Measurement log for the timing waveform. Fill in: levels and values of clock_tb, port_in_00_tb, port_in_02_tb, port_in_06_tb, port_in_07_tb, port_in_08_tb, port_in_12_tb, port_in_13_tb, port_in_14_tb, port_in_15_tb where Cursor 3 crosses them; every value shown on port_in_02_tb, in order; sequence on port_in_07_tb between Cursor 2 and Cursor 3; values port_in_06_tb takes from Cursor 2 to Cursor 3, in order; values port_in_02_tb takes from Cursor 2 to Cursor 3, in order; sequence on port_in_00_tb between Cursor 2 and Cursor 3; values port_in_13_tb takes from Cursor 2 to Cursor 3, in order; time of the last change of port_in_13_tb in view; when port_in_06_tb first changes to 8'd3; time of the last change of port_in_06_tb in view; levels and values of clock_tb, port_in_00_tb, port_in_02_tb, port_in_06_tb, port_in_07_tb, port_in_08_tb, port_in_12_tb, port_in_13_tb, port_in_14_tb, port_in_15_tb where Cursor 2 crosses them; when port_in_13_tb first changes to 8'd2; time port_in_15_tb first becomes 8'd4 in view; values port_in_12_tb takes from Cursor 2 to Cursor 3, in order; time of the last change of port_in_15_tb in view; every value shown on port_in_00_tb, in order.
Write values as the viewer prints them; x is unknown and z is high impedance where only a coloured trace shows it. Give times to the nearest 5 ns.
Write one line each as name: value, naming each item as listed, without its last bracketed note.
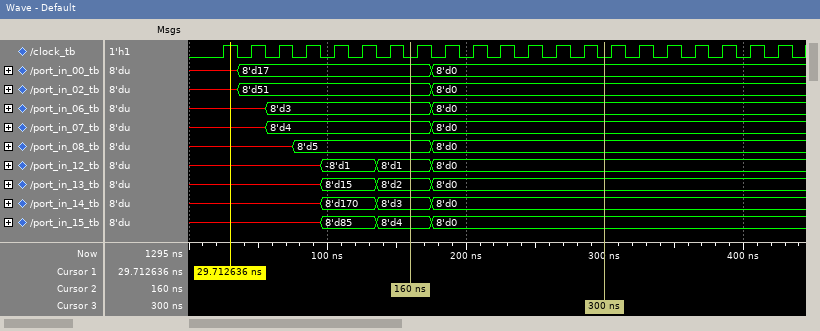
levels and values of clock_tb, port_in_00_tb, port_in_02_tb, port_in_06_tb, port_in_07_tb, port_in_08_tb, port_in_12_tb, port_in_13_tb, port_in_14_tb, port_in_15_tb where Cursor 3 crosses them: clock_tb=0, port_in_00_tb=8'd0, port_in_02_tb=8'd0, port_in_06_tb=8'd0, port_in_07_tb=8'd0, port_in_08_tb=8'd0, port_in_12_tb=8'd0, port_in_13_tb=8'd0, port_in_14_tb=8'd0, port_in_15_tb=8'd0
every value shown on port_in_02_tb, in order: x, 8'd51, 8'd0
sequence on port_in_07_tb between Cursor 2 and Cursor 3: 8'd4, 8'd0
values port_in_06_tb takes from Cursor 2 to Cursor 3, in order: 8'd3, 8'd0
values port_in_02_tb takes from Cursor 2 to Cursor 3, in order: 8'd51, 8'd0
sequence on port_in_00_tb between Cursor 2 and Cursor 3: 8'd17, 8'd0
values port_in_13_tb takes from Cursor 2 to Cursor 3, in order: 8'd2, 8'd0
time of the last change of port_in_13_tb in view: 175 ns
when port_in_06_tb first changes to 8'd3: 55 ns
time of the last change of port_in_06_tb in view: 175 ns
levels and values of clock_tb, port_in_00_tb, port_in_02_tb, port_in_06_tb, port_in_07_tb, port_in_08_tb, port_in_12_tb, port_in_13_tb, port_in_14_tb, port_in_15_tb where Cursor 2 crosses them: clock_tb=0, port_in_00_tb=8'd17, port_in_02_tb=8'd51, port_in_06_tb=8'd3, port_in_07_tb=8'd4, port_in_08_tb=8'd5, port_in_12_tb=8'd1, port_in_13_tb=8'd2, port_in_14_tb=8'd3, port_in_15_tb=8'd4
when port_in_13_tb first changes to 8'd2: 135 ns
time port_in_15_tb first becomes 8'd4 in view: 135 ns
values port_in_12_tb takes from Cursor 2 to Cursor 3, in order: 8'd1, 8'd0
time of the last change of port_in_15_tb in view: 175 ns
every value shown on port_in_00_tb, in order: x, 8'd17, 8'd0
